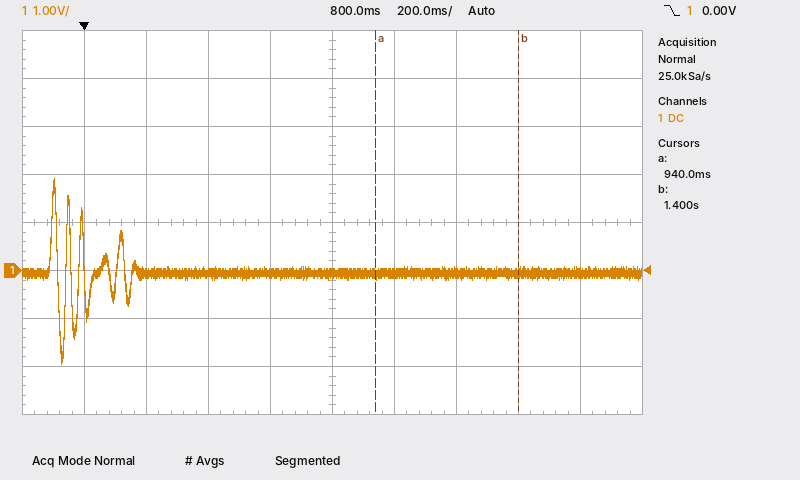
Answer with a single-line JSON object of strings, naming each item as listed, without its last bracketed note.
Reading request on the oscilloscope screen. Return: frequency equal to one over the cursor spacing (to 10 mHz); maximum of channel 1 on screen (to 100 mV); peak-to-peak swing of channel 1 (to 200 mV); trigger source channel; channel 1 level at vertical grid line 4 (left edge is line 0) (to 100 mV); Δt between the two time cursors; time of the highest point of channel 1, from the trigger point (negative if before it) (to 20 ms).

{"frequency equal to one over the cursor spacing": "2.17 Hz", "maximum of channel 1 on screen": "1.9 V", "peak-to-peak swing of channel 1": "3.8 V", "trigger source channel": "channel 1", "channel 1 level at vertical grid line 4 (left edge is line 0)": "-100 mV", "Δt between the two time cursors": "460 ms", "time of the highest point of channel 1, from the trigger point (negative if before it)": "-100 ms"}
